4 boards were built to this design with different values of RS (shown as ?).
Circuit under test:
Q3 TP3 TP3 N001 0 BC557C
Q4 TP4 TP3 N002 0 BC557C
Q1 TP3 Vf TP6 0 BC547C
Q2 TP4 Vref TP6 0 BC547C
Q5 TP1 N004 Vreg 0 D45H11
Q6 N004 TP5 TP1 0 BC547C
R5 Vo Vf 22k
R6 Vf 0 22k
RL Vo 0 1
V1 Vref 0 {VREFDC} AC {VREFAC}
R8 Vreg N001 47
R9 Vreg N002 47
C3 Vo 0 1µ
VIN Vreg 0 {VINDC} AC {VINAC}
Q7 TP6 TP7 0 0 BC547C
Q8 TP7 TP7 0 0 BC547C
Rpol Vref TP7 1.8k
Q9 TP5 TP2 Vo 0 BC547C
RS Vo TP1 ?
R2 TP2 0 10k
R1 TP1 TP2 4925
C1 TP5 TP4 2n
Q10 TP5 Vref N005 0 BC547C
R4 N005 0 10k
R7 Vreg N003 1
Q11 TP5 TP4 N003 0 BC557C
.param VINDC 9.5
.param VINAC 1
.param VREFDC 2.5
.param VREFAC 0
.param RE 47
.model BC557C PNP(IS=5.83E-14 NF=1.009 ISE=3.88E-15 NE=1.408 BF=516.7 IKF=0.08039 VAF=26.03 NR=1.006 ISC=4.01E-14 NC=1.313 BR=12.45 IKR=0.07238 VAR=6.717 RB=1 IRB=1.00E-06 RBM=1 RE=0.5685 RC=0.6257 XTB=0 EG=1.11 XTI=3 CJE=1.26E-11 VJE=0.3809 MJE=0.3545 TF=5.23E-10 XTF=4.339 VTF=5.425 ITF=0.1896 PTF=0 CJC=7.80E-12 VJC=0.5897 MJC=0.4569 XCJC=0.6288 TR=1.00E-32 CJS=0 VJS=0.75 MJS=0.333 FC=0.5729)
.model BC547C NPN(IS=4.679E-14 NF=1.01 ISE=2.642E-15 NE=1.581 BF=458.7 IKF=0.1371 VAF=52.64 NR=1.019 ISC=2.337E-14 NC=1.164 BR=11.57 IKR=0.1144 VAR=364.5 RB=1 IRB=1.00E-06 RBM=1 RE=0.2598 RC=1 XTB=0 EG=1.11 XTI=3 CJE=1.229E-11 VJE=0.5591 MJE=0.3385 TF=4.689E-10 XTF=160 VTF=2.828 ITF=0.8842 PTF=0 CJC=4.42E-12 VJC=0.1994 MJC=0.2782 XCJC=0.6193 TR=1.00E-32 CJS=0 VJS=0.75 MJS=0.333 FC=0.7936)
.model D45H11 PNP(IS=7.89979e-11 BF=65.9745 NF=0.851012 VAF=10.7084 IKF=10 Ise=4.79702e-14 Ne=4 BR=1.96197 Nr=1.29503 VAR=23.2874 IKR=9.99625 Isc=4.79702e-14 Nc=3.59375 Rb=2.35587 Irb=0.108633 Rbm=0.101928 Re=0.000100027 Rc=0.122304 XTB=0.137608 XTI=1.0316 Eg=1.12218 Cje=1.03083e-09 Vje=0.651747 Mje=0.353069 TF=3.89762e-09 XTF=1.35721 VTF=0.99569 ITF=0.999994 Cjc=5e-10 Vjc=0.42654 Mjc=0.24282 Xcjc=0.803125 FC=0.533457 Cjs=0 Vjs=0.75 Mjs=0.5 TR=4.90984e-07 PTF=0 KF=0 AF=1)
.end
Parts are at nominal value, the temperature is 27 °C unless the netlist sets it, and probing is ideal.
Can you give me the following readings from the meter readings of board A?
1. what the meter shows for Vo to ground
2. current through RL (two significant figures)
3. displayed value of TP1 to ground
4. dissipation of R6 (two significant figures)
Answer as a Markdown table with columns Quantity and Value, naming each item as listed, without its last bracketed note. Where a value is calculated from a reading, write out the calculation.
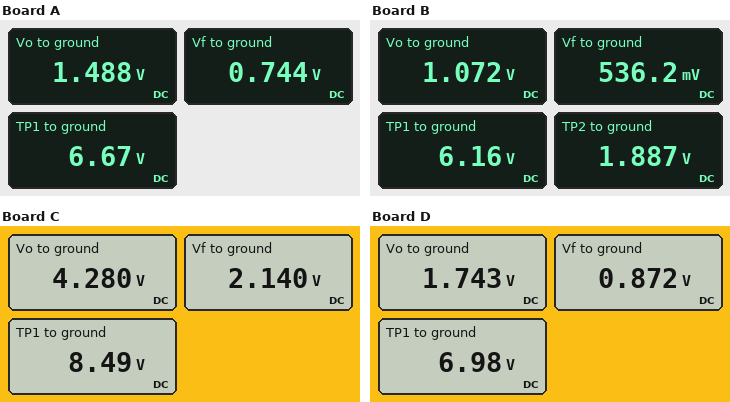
| Quantity | Value |
|---|---|
| what the meter shows for Vo to ground | 1.488 V |
| current through RL | (1.488 V) / 1 Ω = 1.5 A |
| displayed value of TP1 to ground | 6.67 V |
| dissipation of R6 | (744 mV)^2 / 22 kΩ = 25 µW |
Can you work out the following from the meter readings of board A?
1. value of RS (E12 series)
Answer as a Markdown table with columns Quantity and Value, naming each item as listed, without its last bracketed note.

| Quantity | Value |
|---|---|
| value of RS | 3.9 Ω |
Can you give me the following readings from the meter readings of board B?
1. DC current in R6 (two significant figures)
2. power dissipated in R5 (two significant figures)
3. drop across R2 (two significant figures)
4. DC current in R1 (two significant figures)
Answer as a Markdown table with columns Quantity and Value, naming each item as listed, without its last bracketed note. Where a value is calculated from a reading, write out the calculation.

| Quantity | Value |
|---|---|
| DC current in R6 | (536.2 mV) / 22 kΩ = 24 µA |
| power dissipated in R5 | (1.072 V - 536.2 mV)^2 / 22 kΩ = 13 µW |
| drop across R2 | 1.887 V = 1.9 V |
| DC current in R1 | (6.16 V - 1.887 V) / 4.925 kΩ = 870 µA |
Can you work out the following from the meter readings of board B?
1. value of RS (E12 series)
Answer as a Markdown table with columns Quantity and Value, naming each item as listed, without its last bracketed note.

| Quantity | Value |
|---|---|
| value of RS | 5.6 Ω |
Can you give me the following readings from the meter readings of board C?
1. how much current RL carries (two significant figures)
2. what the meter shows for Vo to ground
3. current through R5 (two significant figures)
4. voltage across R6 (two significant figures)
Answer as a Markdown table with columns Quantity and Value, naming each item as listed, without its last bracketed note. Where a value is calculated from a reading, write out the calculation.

| Quantity | Value |
|---|---|
| how much current RL carries | (4.28 V) / 1 Ω = 4.3 A |
| what the meter shows for Vo to ground | 4.280 V |
| current through R5 | (4.28 V - 2.14 V) / 22 kΩ = 97 µA |
| voltage across R6 | 2.14 V = 2.1 V |
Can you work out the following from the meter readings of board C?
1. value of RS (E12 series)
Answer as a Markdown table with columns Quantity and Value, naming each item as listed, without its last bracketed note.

| Quantity | Value |
|---|---|
| value of RS | 1 Ω |
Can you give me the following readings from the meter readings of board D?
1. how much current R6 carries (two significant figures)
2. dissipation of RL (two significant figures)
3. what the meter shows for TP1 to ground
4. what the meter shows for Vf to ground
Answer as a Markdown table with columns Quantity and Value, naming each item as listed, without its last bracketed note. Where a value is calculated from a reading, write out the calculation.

| Quantity | Value |
|---|---|
| how much current R6 carries | (872 mV) / 22 kΩ = 40 µA |
| dissipation of RL | (1.743 V)^2 / 1 Ω = 3.0 W |
| what the meter shows for TP1 to ground | 6.98 V |
| what the meter shows for Vf to ground | 0.872 V |
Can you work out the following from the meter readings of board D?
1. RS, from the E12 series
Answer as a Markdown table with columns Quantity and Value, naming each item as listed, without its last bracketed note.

| Quantity | Value |
|---|---|
| RS, from the E12 series | 3.3 Ω |
